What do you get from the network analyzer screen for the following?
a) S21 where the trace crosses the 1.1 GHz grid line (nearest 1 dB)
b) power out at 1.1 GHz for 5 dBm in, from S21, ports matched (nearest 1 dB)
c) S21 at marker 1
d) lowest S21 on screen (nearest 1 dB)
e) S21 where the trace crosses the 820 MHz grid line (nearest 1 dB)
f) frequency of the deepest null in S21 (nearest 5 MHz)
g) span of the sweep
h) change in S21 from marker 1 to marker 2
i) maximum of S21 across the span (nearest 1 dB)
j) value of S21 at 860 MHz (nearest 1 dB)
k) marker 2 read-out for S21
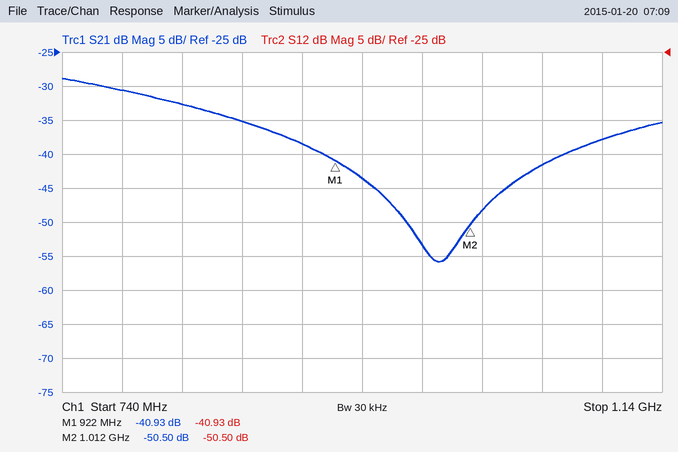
-38 dB
-33 dBm
-40.93 dB
-56 dB
-33 dB
990 MHz
400 MHz
-9.57 dB
-29 dB
-35 dB
-50.50 dB
